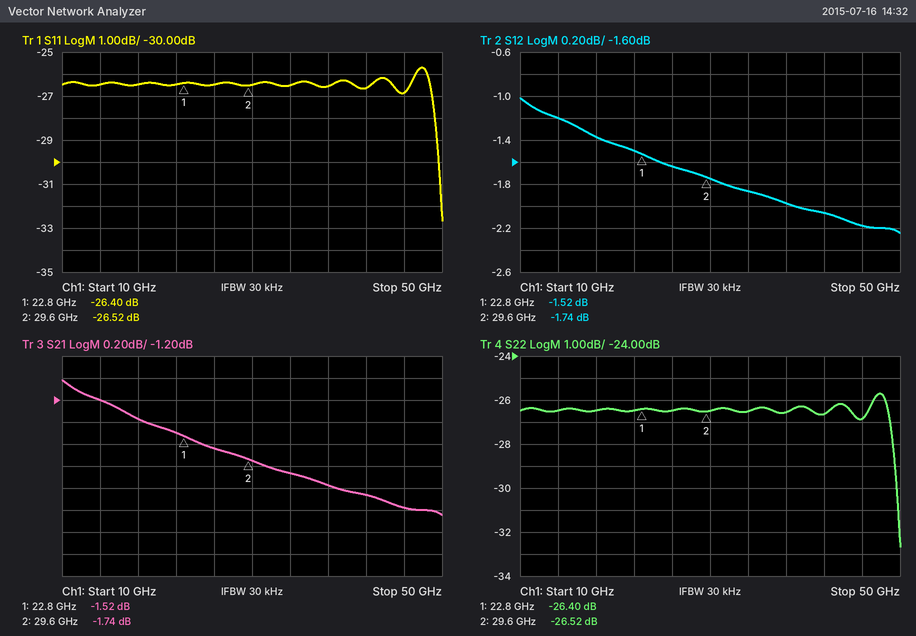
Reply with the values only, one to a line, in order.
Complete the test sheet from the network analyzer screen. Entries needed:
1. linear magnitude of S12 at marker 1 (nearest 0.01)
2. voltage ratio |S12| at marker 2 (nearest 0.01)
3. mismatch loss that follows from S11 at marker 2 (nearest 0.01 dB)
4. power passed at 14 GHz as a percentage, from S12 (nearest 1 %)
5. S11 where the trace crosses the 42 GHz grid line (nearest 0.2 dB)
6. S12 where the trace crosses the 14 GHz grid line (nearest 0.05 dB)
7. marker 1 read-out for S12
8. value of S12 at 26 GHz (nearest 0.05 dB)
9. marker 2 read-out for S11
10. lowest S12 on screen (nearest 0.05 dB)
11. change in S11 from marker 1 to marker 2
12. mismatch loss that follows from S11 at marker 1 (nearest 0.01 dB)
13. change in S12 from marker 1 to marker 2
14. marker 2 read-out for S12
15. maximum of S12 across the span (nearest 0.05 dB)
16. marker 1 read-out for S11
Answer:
0.84
0.82
0.01 dB
76 %
-26.6 dB
-1.20 dB
-1.52 dB
-1.65 dB
-26.52 dB
-2.25 dB
-0.12 dB
0.01 dB
-0.22 dB
-1.74 dB
-1.00 dB
-26.40 dB
